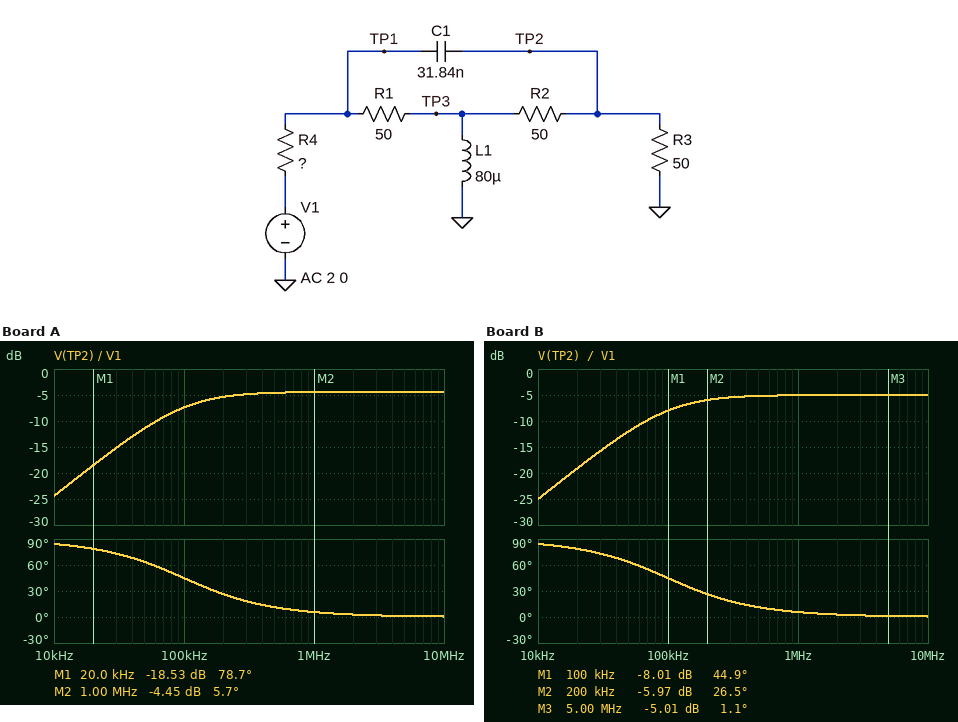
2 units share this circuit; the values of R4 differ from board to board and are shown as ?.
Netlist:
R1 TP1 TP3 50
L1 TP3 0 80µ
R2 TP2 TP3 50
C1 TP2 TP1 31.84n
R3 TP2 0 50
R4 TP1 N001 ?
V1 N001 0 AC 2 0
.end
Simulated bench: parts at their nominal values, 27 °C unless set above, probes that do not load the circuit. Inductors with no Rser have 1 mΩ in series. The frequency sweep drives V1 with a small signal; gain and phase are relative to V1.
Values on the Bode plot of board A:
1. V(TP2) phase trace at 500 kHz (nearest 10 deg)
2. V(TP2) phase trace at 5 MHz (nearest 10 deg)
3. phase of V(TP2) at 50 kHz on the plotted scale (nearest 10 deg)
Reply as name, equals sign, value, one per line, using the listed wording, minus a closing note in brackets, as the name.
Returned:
V(TP2) phase trace at 500 kHz = 10 deg
V(TP2) phase trace at 5 MHz = 0 deg
phase of V(TP2) at 50 kHz on the plotted scale = 60 deg
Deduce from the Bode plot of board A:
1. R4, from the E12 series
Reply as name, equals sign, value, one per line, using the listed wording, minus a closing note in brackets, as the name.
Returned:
R4, from the E12 series = 33 Ω
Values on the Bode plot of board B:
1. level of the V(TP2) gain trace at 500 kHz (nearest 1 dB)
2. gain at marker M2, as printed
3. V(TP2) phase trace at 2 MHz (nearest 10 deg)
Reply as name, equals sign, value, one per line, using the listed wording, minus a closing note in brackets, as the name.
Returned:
level of the V(TP2) gain trace at 500 kHz = -5 dB
gain at marker M2, as printed = -5.97 dB
V(TP2) phase trace at 2 MHz = 0 deg
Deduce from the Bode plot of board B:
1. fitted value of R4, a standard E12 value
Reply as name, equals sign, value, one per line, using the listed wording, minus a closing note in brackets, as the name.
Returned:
fitted value of R4, a standard E12 value = 39 Ω
